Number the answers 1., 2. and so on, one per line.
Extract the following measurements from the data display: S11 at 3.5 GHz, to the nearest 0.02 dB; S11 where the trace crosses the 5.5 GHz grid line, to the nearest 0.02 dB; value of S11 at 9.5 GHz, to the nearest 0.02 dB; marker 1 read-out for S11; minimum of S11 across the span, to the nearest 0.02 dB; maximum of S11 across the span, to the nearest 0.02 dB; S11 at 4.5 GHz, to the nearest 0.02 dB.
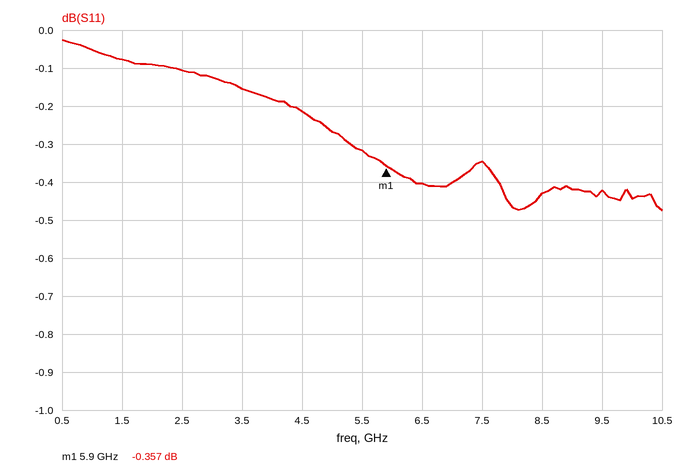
1. -0.16 dB
2. -0.32 dB
3. -0.42 dB
4. -0.357 dB
5. -0.48 dB
6. -0.02 dB
7. -0.22 dB
